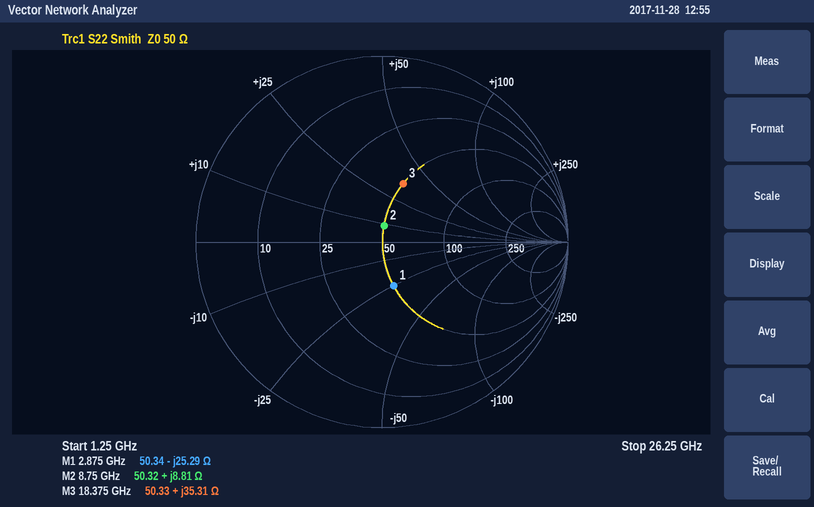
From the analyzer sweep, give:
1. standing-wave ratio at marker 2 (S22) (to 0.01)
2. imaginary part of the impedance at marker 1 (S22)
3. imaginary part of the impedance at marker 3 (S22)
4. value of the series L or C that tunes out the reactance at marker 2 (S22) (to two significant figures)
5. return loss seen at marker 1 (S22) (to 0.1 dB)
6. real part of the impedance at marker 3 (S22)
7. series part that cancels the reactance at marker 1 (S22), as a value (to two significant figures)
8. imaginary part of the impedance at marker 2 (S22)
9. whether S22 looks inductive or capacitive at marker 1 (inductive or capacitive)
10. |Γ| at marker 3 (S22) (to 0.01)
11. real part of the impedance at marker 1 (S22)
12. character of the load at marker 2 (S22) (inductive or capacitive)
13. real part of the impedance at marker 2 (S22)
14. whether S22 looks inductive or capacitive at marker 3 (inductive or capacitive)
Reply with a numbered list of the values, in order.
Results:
1. 1.19
2. -25.29 Ω
3. +35.31 Ω
4. 2.1 pF
5. 12.2 dB
6. 50.33 Ω
7. 1.4 nH
8. +8.81 Ω
9. capacitive
10. 0.33
11. 50.34 Ω
12. inductive
13. 50.32 Ω
14. inductive
